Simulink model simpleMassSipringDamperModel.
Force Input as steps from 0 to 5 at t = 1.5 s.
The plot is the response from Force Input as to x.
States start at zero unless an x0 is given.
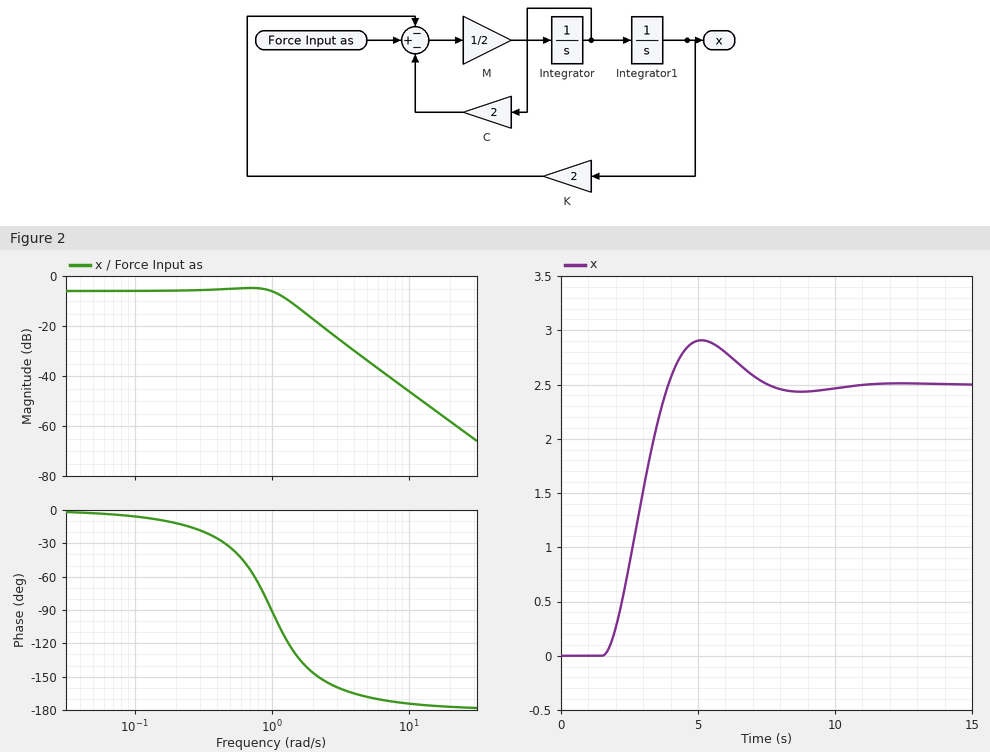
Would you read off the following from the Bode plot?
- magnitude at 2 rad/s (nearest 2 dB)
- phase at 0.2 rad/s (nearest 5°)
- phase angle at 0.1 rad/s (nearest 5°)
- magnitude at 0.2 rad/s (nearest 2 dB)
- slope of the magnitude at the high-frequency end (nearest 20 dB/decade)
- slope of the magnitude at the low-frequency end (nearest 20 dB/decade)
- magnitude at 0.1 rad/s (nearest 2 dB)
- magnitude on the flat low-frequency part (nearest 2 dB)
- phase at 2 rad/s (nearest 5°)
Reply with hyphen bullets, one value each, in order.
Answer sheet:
- -18 dB
- -10°
- -5°
- -6 dB
- -40 dB/decade
- 0 dB/decade
- -6 dB
- -6 dB
- -145°
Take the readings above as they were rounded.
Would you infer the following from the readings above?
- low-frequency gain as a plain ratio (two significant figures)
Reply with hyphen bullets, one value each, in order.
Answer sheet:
- 0.50
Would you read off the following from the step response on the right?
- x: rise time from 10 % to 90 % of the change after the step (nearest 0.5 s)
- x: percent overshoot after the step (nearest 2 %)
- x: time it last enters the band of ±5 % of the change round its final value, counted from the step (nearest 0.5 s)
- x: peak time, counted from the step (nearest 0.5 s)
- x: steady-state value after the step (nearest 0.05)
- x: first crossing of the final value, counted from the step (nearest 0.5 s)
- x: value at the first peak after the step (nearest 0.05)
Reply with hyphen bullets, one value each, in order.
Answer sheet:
- 1.5 s
- 16 %
- 5.5 s
- 3.5 s
- 2.50
- 2.5 s
- 2.90
